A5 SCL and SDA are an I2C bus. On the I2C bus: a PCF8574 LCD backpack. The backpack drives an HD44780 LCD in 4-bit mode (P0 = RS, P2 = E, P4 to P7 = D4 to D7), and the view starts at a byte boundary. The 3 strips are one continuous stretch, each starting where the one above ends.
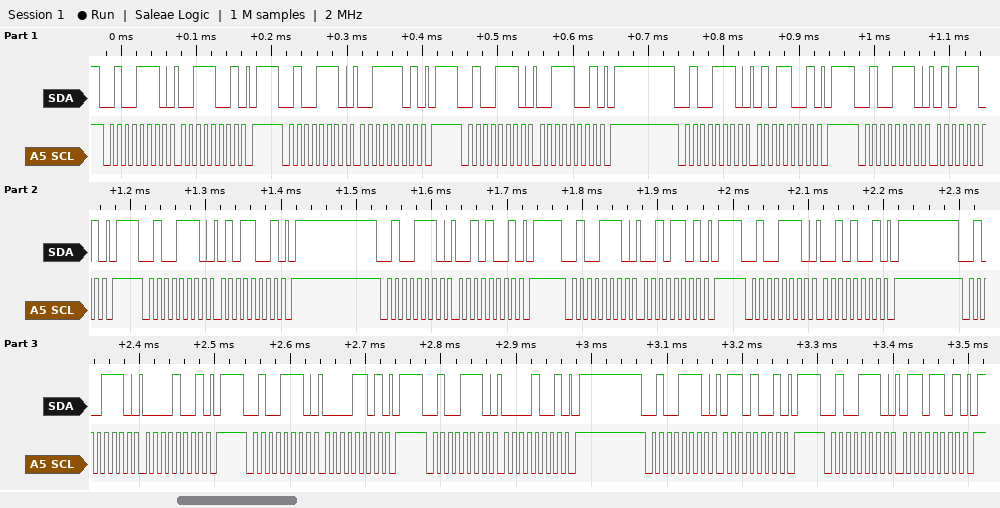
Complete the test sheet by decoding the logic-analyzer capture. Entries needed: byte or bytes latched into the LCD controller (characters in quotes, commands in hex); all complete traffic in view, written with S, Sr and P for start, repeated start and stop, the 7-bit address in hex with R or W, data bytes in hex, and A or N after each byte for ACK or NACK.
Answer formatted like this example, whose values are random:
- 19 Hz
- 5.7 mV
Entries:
- '5' ' '
- S 27W A 39 A P S 27W A 3D A P S 27W A 39 A P S 27W A 59 A P S 27W A 5D A P S 27W A 59 A P S 27W A 29 A P S 27W A 2D A P S 27W A 29 A P S 27W A 09 A P S 27W A 0D A P S 27W A 09 A P S 27W A 69 A P S 27W A 6D A P
